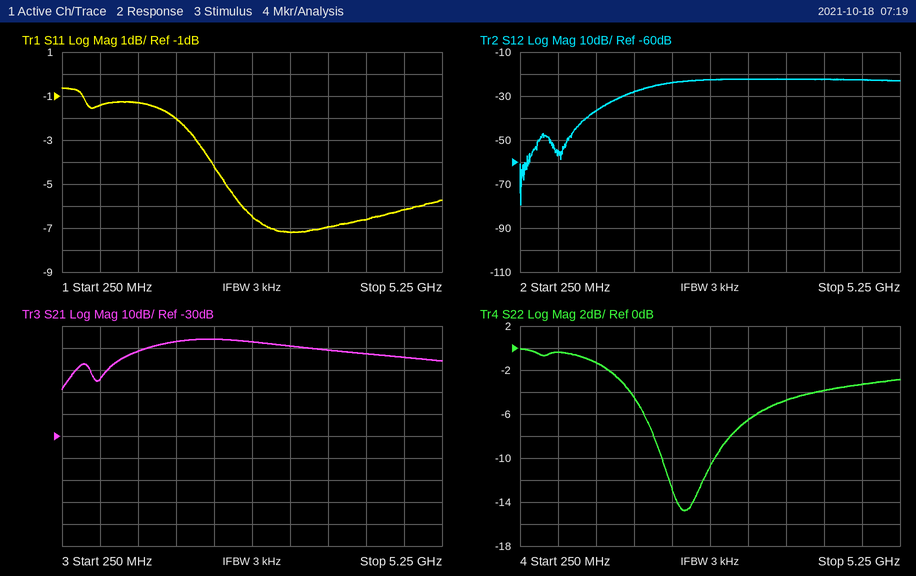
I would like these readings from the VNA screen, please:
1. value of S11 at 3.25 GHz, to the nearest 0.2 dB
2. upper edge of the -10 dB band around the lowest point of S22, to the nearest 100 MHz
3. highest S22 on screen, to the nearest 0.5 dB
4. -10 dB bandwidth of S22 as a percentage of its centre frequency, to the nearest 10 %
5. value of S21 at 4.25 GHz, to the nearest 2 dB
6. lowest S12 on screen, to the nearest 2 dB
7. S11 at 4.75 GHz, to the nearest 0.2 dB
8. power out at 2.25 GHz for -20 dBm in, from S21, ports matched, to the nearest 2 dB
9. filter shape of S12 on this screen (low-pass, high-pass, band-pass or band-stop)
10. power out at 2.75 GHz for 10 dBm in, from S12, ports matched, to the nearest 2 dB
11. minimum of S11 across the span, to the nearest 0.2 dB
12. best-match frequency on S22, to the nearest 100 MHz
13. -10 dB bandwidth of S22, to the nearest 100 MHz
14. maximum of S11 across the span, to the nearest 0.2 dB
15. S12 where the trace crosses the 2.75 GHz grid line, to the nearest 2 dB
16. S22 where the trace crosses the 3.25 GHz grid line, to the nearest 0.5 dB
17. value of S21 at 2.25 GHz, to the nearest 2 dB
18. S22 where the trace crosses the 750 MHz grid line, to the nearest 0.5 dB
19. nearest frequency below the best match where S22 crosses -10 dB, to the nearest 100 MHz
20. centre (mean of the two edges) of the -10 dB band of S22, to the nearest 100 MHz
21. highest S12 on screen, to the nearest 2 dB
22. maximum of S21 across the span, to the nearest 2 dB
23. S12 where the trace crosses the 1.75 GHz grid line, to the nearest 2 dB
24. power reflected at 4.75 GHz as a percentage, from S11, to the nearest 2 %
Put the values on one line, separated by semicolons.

-7.2 dB; 2.8 GHz; 0.0 dB; 30 %; 8 dB; -80 dB; -6.2 dB; -6 dBm; high-pass; -12 dBm; -7.2 dB; 2.4 GHz; 700 MHz; -0.6 dB; -22 dB; -6.5 dB; 14 dB; -0.5 dB; 2.1 GHz; 2.5 GHz; -22 dB; 14 dB; -28 dB; 24 %
